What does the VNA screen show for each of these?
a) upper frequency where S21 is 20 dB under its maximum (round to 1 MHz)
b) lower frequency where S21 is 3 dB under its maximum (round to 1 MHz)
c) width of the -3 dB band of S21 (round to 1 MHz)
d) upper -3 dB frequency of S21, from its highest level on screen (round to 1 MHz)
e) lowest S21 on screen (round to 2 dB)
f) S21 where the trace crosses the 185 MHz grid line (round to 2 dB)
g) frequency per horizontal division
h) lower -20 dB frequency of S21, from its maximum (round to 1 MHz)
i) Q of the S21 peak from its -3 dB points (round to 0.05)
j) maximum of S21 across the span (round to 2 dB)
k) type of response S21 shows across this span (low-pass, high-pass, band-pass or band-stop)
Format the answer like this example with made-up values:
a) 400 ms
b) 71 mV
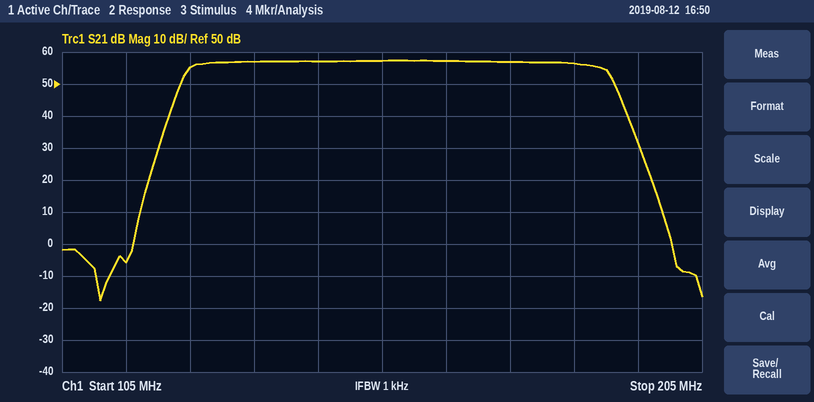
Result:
a) 194 MHz
b) 125 MHz
c) 65 MHz
d) 190 MHz
e) -18 dB
f) 56 dB
g) 10 MHz
h) 121 MHz
i) 2.40
j) 58 dB
k) band-pass
